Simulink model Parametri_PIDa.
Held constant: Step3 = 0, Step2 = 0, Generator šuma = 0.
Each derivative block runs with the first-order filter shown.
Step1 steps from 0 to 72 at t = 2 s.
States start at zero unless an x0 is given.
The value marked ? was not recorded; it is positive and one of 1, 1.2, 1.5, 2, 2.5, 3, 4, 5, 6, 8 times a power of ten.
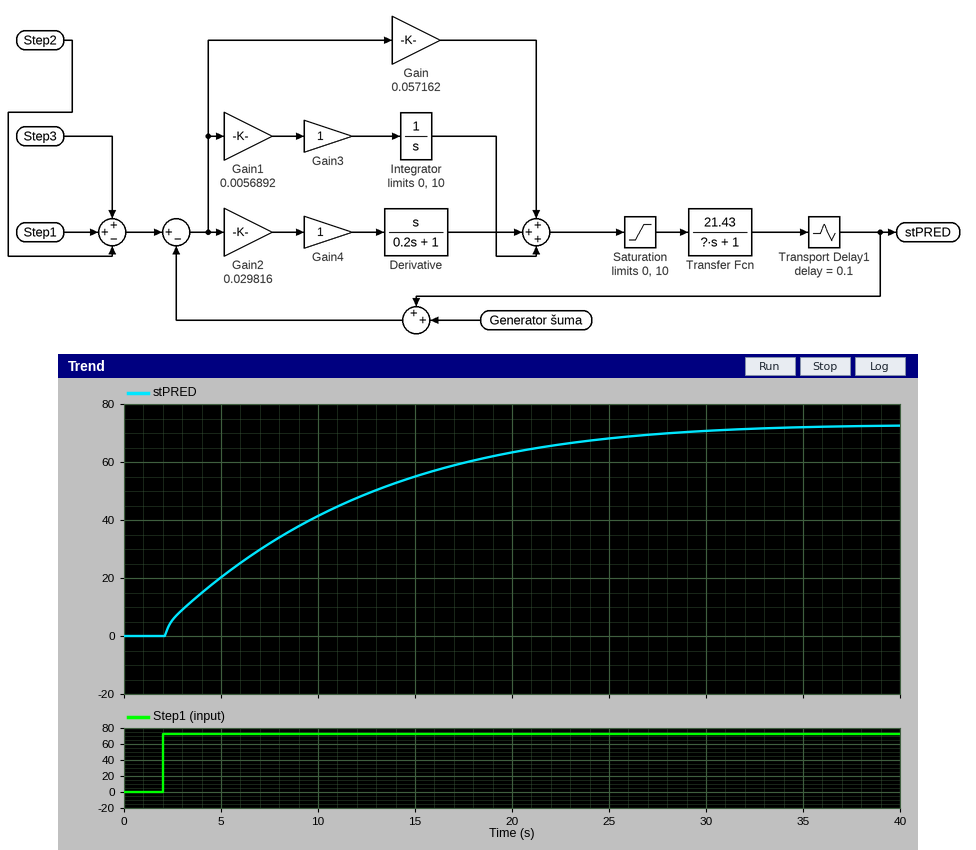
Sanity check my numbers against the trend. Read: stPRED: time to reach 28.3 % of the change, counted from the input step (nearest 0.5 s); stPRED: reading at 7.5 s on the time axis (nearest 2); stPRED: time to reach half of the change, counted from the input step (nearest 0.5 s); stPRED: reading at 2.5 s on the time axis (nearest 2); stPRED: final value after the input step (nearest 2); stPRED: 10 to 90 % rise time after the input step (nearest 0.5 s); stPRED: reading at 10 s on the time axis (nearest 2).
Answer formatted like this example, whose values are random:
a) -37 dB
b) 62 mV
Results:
a) 3.0 s
b) 32
c) 6.5 s
d) 6
e) 72
f) 18.5 s
g) 42
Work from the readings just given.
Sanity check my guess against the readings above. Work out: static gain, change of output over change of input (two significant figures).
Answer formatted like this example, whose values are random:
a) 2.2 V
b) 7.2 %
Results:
a) 1.0
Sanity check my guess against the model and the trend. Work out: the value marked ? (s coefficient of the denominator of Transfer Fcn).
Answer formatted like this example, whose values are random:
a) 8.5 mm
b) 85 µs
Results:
a) 12
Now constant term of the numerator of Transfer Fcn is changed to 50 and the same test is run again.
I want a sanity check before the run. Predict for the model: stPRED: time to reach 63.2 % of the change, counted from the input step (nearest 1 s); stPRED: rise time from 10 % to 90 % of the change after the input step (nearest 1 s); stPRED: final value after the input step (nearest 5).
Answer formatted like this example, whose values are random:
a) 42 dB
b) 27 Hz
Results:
a) 4 s
b) 9 s
c) 70
